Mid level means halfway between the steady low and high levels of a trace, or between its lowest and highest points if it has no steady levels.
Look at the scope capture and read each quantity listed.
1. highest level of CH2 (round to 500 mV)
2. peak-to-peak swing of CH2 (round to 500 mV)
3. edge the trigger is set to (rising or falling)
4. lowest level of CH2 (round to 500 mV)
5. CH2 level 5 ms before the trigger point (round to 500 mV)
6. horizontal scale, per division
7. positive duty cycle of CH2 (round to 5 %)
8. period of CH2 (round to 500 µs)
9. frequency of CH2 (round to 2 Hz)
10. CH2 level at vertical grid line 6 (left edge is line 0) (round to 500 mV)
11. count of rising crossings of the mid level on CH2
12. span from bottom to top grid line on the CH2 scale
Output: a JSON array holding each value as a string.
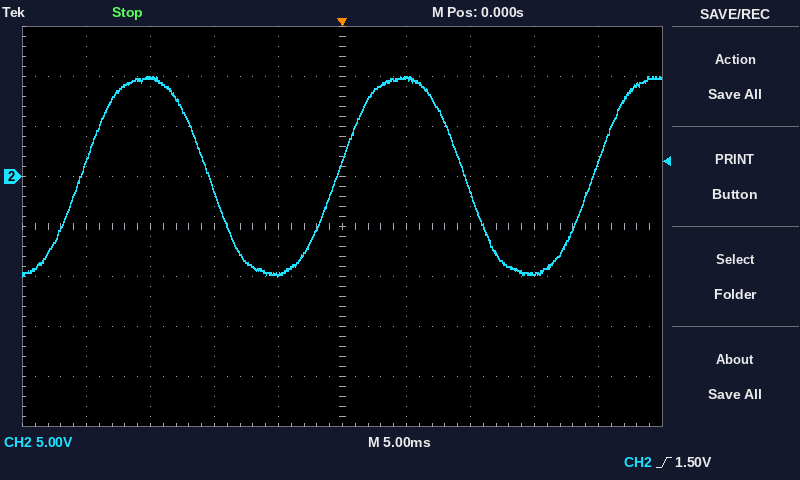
["10.0 V", "20.0 V", "rising", "-10.0 V", "-10.0 V", "5 ms", "50 %", "20.0 ms", "50 Hz", "10.0 V", "3", "40 V"]
